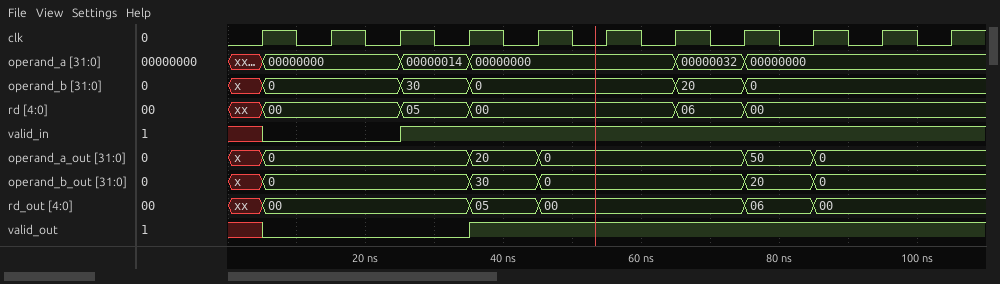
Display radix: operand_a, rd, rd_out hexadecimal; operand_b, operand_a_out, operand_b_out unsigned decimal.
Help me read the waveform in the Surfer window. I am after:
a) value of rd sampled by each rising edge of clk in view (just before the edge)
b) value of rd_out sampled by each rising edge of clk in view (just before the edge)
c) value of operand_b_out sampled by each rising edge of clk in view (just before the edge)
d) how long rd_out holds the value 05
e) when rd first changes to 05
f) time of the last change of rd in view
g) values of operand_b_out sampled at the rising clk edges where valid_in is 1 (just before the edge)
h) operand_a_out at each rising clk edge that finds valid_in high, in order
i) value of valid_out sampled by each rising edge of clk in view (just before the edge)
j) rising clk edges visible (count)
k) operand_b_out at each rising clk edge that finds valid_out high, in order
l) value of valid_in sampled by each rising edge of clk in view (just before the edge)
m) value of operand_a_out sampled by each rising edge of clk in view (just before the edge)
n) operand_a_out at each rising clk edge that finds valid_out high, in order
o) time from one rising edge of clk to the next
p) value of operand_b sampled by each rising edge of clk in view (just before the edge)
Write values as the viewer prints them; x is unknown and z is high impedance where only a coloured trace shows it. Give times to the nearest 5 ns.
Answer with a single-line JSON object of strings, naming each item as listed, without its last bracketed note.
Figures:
{"value of rd sampled by each rising edge of clk in view": "xx, 00, 00, 05, 00, 00, 00, 06, 00, 00, 00", "value of rd_out sampled by each rising edge of clk in view": "xx, 00, 00, 00, 05, 00, 00, 00, 06, 00, 00", "value of operand_b_out sampled by each rising edge of clk in view": "x, 0, 0, 0, 30, 0, 0, 0, 20, 0, 0", "how long rd_out holds the value 05": "10 ns", "when rd first changes to 05": "25 ns", "time of the last change of rd in view": "75 ns", "values of operand_b_out sampled at the rising clk edges where valid_in is 1": "0, 30, 0, 0, 0, 20, 0, 0", "operand_a_out at each rising clk edge that finds valid_in high, in order": "0, 20, 0, 0, 0, 50, 0, 0", "value of valid_out sampled by each rising edge of clk in view": "x 0 0 0 1 1 1 1 1 1 1", "rising clk edges visible": "11", "operand_b_out at each rising clk edge that finds valid_out high, in order": "30, 0, 0, 0, 20, 0, 0", "value of valid_in sampled by each rising edge of clk in view": "x 0 0 1 1 1 1 1 1 1 1", "value of operand_a_out sampled by each rising edge of clk in view": "x, 0, 0, 0, 20, 0, 0, 0, 50, 0, 0", "operand_a_out at each rising clk edge that finds valid_out high, in order": "20, 0, 0, 0, 50, 0, 0", "time from one rising edge of clk to the next": "10 ns", "value of operand_b sampled by each rising edge of clk in view": "x, 0, 0, 30, 0, 0, 0, 20, 0, 0, 0"}
